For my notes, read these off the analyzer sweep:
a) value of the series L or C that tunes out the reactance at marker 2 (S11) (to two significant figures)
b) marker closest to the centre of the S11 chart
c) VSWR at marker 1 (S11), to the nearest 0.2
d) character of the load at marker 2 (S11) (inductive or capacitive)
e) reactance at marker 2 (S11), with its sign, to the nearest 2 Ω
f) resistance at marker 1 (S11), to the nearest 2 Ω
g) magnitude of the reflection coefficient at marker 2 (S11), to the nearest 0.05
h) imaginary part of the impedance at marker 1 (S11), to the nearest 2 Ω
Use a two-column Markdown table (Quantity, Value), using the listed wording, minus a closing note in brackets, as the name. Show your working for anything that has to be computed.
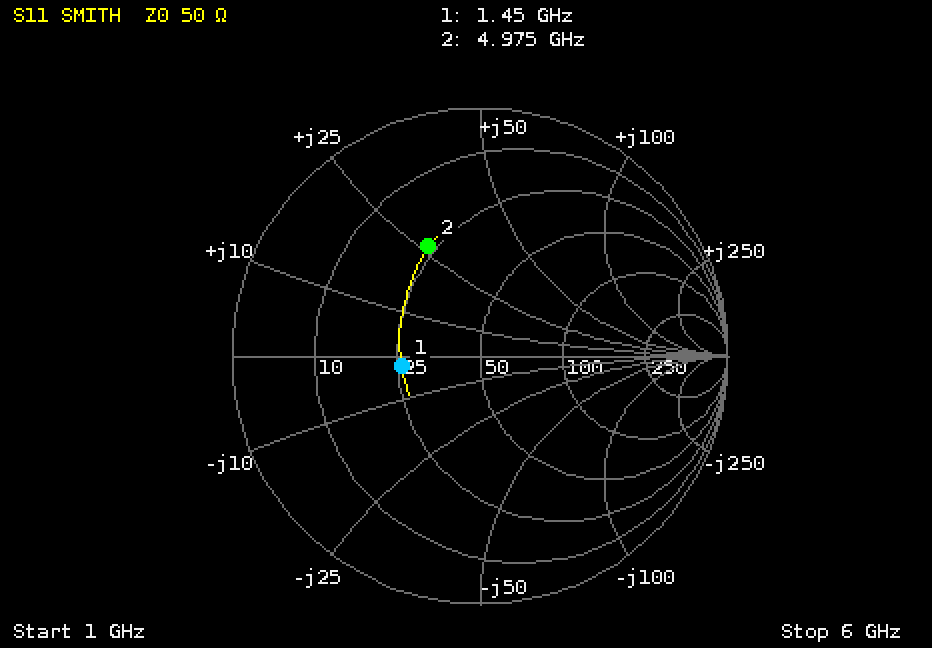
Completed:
| Quantity | Value |
|---|---|
| value of the series L or C that tunes out the reactance at marker 2 (S11) | C = 1/(2π × 4.975 GHz × 26 Ω) ≈ 1.2 pF |
| marker closest to the centre of the S11 chart | marker 1 |
| VSWR at marker 1 (S11), to the nearest 0.2 | 2.0 |
| character of the load at marker 2 (S11) | inductive |
| reactance at marker 2 (S11), with its sign, to the nearest 2 Ω | +26 Ω |
| resistance at marker 1 (S11), to the nearest 2 Ω | 26 Ω |
| magnitude of the reflection coefficient at marker 2 (S11), to the nearest 0.05 | 0.50 |
| imaginary part of the impedance at marker 1 (S11), to the nearest 2 Ω | -2 Ω |
